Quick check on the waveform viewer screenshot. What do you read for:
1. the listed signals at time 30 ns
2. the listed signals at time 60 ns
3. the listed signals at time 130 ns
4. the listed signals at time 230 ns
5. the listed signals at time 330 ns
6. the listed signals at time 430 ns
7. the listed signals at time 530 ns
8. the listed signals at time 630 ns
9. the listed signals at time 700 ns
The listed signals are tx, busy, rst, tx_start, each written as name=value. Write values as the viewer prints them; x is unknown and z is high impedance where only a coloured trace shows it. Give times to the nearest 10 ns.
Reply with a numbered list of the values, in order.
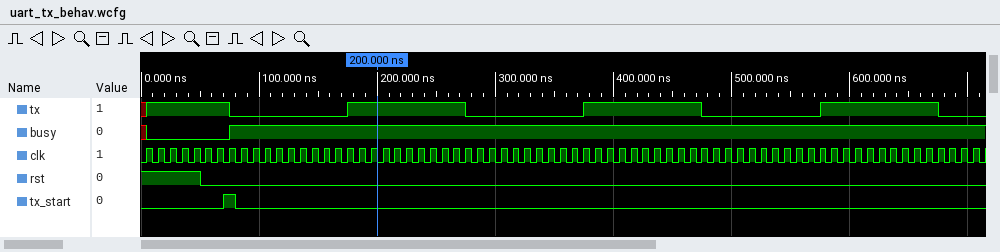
1. tx=1, busy=0, rst=1, tx_start=0
2. tx=1, busy=0, rst=0, tx_start=0
3. tx=0, busy=1, rst=0, tx_start=0
4. tx=1, busy=1, rst=0, tx_start=0
5. tx=0, busy=1, rst=0, tx_start=0
6. tx=1, busy=1, rst=0, tx_start=0
7. tx=0, busy=1, rst=0, tx_start=0
8. tx=1, busy=1, rst=0, tx_start=0
9. tx=0, busy=1, rst=0, tx_start=0
